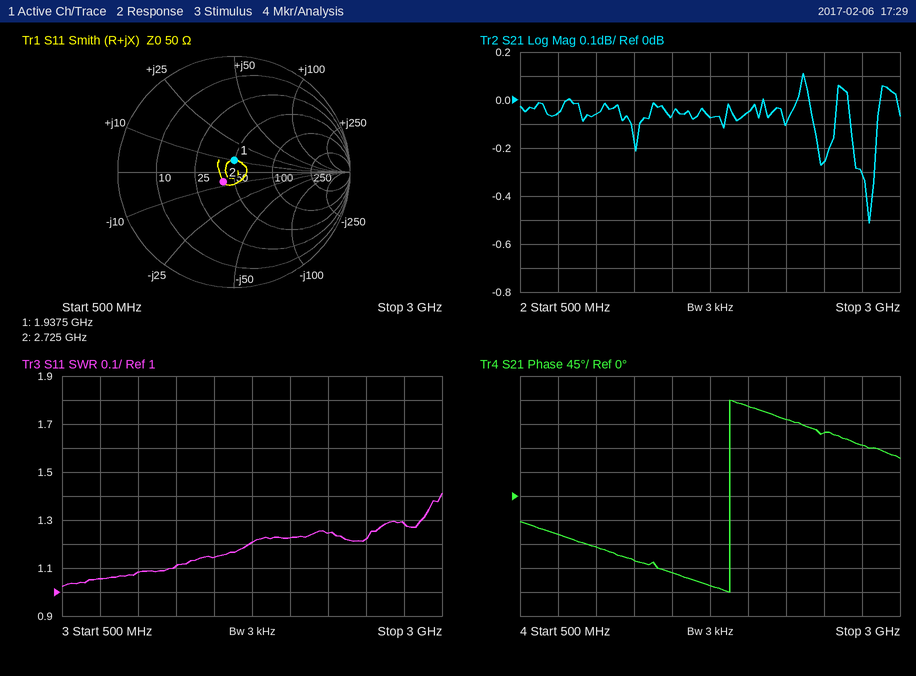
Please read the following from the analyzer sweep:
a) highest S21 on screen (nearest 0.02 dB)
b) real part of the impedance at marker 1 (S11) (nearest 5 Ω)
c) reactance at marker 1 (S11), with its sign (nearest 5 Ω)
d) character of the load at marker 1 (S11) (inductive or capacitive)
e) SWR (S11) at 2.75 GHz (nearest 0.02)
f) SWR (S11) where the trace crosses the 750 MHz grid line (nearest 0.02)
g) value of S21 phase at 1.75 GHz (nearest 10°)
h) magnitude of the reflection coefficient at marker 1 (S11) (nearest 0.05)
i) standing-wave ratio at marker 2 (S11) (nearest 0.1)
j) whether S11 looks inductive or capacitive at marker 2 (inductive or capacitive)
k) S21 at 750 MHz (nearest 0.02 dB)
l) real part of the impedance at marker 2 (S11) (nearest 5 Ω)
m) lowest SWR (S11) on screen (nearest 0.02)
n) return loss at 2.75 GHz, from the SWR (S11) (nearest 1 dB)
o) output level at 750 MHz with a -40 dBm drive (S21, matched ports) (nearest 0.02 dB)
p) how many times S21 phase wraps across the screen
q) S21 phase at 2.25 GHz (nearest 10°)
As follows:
0.12 dB
50 Ω
+10 Ω
inductive
1.28
1.06
-170°
0.10
1.3
capacitive
-0.06 dB
40 Ω
1.02
18 dB
-40.06 dBm
1
140°
